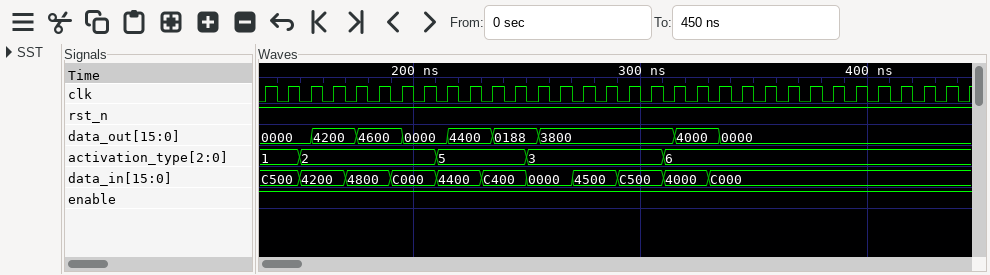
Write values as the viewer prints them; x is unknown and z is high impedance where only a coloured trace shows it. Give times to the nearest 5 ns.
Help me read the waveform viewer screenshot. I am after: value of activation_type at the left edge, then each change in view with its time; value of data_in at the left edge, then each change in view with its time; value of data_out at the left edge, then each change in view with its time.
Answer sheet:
1, 2 at 150 ns, 5 at 210 ns, 3 at 250 ns, 6 at 310 ns
C500, 4200 at 150 ns, 4800 at 170 ns, C000 at 190 ns, 4400 at 210 ns, C400 at 230 ns, 0000 at 250 ns, 4500 at 270 ns, C500 at 290 ns, 4000 at 310 ns, C000 at 330 ns
0000, 4200 at 155 ns, 4600 at 175 ns, 0000 at 195 ns, 4400 at 215 ns, 0188 at 235 ns, 3800 at 255 ns, 4000 at 315 ns, 0000 at 335 ns
